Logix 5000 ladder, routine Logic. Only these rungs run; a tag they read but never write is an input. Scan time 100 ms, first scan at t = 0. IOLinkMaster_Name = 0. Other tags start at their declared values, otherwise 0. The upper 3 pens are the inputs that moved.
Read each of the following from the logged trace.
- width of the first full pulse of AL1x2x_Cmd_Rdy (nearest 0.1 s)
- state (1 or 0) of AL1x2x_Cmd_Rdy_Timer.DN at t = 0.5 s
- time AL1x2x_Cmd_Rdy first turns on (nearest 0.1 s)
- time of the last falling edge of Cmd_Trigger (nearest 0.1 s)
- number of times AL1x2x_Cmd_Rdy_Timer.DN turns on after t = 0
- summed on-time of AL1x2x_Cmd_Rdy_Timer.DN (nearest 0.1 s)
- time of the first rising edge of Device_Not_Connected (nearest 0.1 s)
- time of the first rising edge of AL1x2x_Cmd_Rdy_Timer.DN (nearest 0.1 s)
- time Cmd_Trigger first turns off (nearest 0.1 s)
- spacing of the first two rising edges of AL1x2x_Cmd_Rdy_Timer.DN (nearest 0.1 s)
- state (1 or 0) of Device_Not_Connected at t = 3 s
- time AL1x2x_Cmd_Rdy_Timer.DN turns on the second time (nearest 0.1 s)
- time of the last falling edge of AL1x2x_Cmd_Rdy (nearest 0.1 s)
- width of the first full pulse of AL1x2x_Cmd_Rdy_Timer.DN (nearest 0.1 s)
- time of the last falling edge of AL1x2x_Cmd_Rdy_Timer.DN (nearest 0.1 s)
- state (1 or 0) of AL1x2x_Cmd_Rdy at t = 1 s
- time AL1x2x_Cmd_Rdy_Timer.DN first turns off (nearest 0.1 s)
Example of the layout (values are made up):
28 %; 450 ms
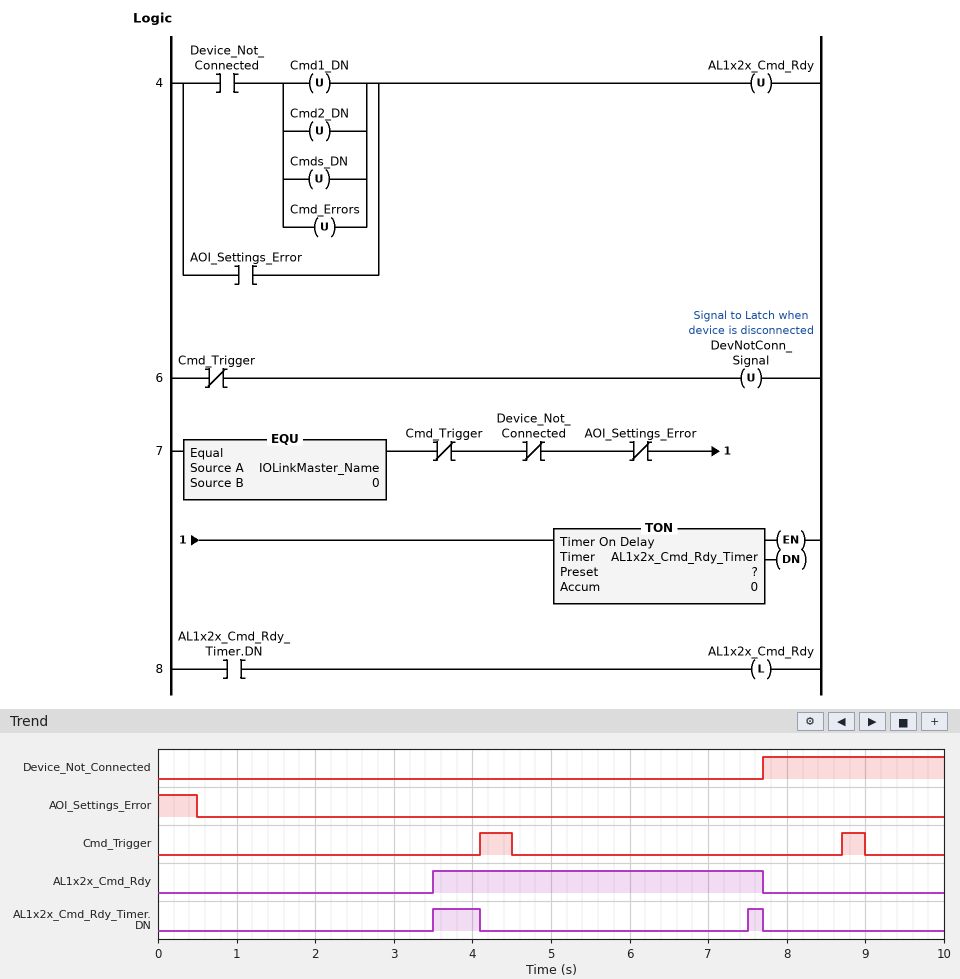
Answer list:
4.2 s; 0; 3.5 s; 9.0 s; 2; 0.8 s; 7.7 s; 3.5 s; 4.5 s; 4.0 s; 0; 7.5 s; 7.7 s; 0.6 s; 7.7 s; 0; 4.1 s
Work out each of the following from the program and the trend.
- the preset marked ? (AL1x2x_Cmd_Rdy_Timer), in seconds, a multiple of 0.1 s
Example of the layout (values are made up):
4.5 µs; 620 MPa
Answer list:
3.0 s
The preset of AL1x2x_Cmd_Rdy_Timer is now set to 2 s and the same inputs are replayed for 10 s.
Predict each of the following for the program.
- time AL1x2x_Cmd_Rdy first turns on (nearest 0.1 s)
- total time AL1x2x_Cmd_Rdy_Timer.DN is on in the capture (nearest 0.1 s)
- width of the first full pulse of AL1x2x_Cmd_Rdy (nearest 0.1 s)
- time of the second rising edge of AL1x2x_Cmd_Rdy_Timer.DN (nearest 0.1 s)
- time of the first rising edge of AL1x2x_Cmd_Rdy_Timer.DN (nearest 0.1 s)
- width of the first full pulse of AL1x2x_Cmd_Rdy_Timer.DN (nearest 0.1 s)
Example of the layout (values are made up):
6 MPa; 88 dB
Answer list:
2.5 s; 2.8 s; 5.2 s; 6.5 s; 2.5 s; 1.6 s
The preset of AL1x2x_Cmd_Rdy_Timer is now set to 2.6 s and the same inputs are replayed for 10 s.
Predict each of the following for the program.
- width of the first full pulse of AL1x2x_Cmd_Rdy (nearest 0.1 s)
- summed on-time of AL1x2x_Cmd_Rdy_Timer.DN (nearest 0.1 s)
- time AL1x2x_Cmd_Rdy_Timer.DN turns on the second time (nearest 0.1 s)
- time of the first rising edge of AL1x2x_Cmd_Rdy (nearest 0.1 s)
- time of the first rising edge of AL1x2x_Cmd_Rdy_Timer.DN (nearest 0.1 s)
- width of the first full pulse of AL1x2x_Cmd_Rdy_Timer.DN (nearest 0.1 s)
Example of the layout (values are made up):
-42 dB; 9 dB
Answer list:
4.6 s; 1.6 s; 7.1 s; 3.1 s; 3.1 s; 1.0 s
